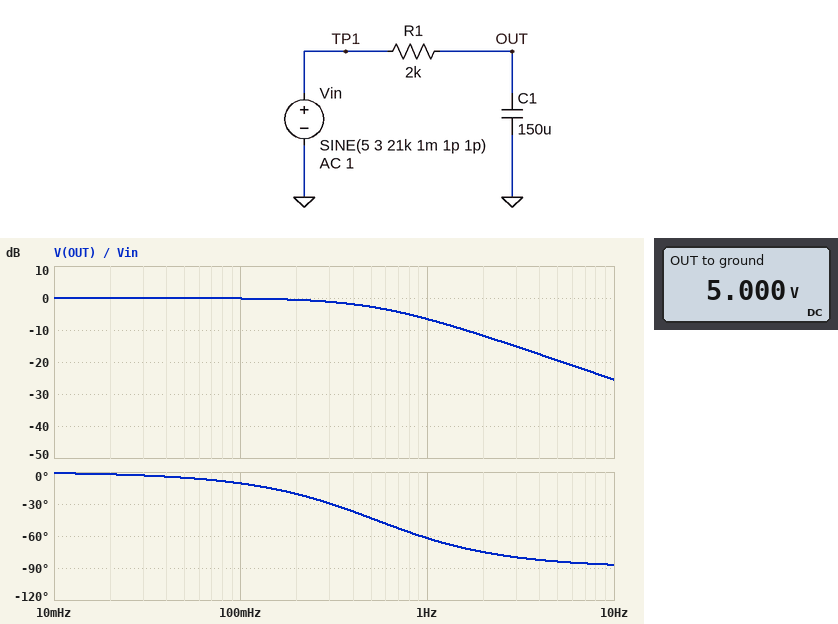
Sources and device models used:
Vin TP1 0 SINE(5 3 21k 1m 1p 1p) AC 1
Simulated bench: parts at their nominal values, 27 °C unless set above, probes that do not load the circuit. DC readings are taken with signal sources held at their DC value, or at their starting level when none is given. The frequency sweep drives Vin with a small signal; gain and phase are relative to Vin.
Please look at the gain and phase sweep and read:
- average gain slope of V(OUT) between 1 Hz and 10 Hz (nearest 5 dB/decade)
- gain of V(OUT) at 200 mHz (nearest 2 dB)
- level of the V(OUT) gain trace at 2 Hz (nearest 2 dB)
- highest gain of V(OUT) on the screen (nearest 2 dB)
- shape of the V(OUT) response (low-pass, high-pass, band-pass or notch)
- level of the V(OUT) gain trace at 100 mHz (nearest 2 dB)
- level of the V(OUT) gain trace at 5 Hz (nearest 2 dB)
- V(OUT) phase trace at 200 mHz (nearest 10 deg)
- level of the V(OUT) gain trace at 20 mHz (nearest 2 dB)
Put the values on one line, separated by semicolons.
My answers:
-20 dB/decade; 0 dB; -12 dB; 0 dB; low-pass; 0 dB; -20 dB; -20 deg; 0 dB
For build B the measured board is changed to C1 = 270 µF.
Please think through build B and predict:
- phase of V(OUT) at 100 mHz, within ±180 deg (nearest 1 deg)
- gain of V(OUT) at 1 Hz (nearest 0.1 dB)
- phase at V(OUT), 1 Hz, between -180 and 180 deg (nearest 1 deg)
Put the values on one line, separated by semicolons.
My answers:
-19 deg; -11.0 dB; -74 deg
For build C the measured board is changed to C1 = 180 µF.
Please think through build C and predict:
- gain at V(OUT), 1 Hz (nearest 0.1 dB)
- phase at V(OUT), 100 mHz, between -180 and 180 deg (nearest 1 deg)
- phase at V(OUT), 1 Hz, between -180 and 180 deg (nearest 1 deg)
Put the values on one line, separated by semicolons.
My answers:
-7.9 dB; -13 deg; -66 deg
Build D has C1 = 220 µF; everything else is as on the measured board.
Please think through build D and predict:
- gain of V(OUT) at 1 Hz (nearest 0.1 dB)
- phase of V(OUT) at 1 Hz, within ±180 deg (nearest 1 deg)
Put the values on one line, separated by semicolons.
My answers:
-9.4 dB; -70 deg
